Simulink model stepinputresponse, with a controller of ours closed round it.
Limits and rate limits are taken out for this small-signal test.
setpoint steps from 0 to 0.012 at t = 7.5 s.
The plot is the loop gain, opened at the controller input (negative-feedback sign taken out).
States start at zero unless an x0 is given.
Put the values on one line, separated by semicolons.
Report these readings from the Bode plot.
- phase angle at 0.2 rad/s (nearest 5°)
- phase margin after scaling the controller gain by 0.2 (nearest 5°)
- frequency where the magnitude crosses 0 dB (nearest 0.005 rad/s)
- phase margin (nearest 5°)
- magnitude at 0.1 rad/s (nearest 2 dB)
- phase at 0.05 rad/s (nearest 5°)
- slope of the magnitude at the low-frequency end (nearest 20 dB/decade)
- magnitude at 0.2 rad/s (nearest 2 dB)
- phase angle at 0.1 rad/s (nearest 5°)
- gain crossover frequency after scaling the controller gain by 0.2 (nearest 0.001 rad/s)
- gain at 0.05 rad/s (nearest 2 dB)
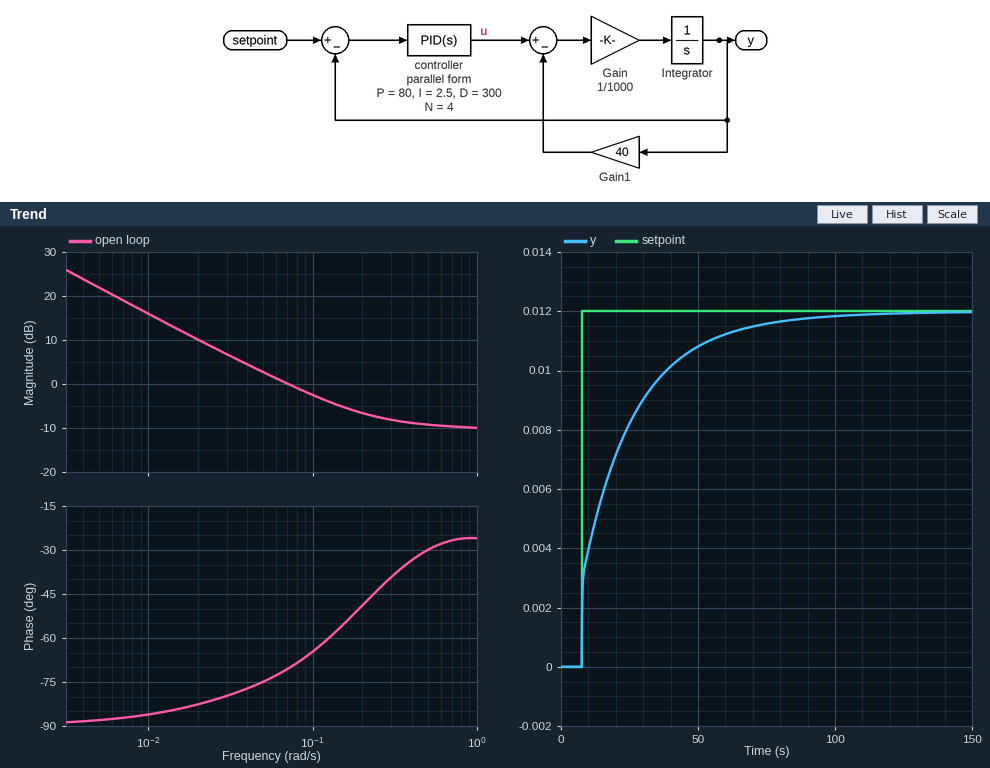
-50°; 95°; 0.070 rad/s; 110°; -2 dB; -75°; -20 dB/decade; -6 dB; -65°; 0.013 rad/s; 2 dB
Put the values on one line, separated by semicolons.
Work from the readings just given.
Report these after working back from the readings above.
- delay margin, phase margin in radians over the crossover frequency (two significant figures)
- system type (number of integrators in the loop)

27 s; 1
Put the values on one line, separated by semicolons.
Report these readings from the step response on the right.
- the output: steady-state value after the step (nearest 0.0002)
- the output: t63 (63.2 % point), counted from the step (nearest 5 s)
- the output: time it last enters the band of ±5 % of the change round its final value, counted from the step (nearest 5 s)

0.0120; 15 s; 60 s
